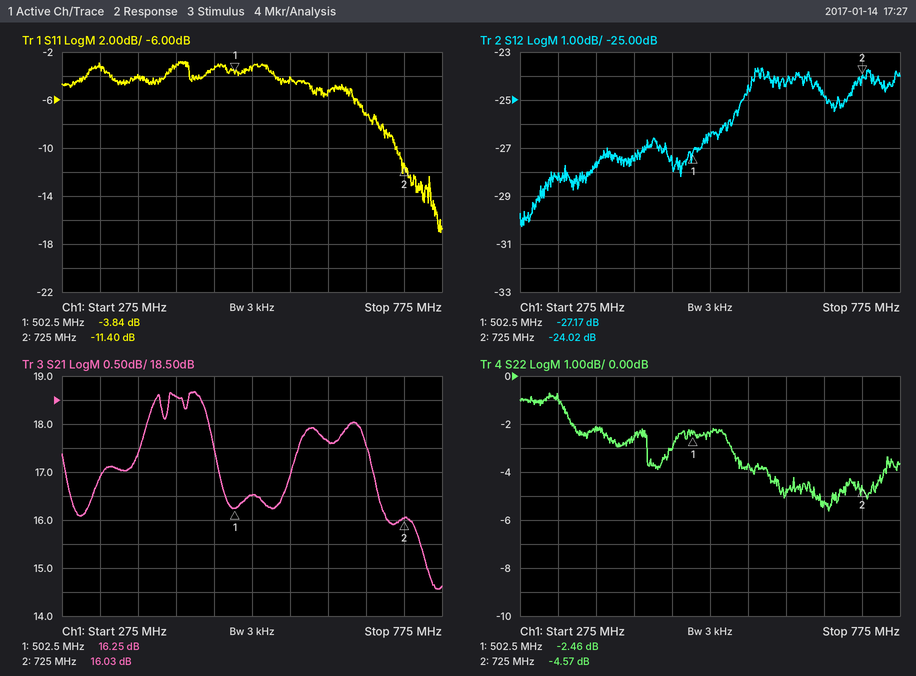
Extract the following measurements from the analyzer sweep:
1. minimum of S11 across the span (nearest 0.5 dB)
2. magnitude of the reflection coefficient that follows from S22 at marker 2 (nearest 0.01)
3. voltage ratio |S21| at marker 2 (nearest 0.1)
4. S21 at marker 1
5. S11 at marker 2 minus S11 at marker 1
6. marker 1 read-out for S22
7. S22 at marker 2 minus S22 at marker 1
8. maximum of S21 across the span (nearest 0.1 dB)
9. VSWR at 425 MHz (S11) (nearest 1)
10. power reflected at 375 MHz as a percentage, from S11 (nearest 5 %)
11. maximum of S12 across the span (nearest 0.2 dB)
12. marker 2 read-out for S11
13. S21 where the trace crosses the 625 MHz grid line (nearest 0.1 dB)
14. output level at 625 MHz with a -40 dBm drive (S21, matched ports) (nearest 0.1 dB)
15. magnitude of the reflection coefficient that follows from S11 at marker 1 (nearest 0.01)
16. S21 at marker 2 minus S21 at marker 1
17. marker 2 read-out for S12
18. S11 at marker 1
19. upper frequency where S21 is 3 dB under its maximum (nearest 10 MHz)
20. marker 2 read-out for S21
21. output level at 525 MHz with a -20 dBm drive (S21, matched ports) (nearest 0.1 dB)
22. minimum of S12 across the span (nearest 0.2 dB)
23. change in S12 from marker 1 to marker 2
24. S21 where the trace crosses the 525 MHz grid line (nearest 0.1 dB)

-17.0 dB
0.59
6.3
16.25 dB
-7.56 dB
-2.46 dB
-2.11 dB
18.7 dB
6
40 %
-23.6 dB
-11.40 dB
17.6 dB
-22.4 dBm
0.64
-0.22 dB
-24.02 dB
-3.84 dB
740 MHz
16.03 dB
-3.5 dBm
-30.2 dB
3.15 dB
16.5 dB
